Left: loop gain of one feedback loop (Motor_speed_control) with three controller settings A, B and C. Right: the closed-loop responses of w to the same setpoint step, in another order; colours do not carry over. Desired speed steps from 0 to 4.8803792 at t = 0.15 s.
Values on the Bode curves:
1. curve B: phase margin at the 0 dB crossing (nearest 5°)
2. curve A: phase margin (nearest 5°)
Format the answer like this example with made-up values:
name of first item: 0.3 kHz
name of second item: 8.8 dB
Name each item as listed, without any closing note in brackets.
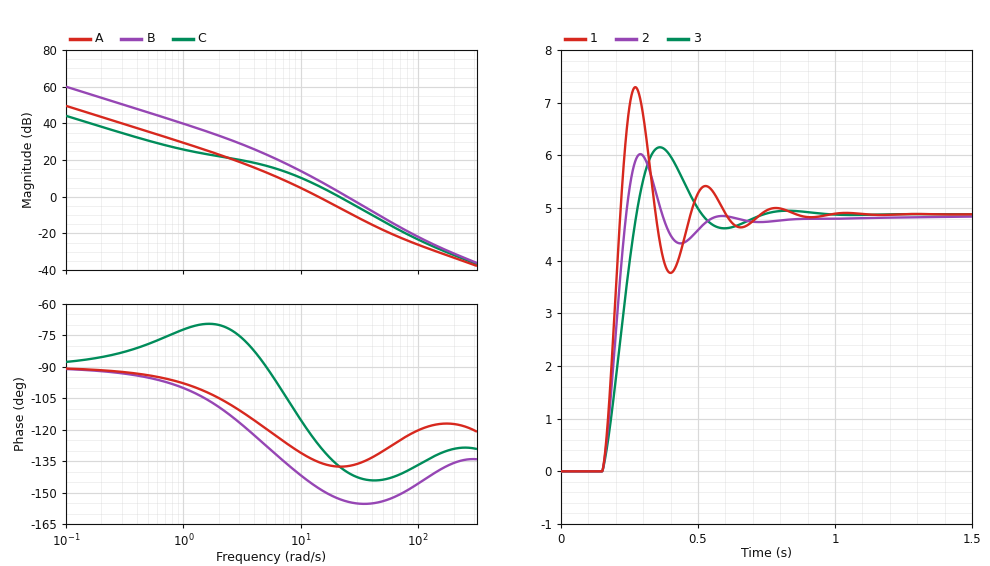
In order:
curve B: phase margin at the 0 dB crossing: 25°
curve A: phase margin: 45°
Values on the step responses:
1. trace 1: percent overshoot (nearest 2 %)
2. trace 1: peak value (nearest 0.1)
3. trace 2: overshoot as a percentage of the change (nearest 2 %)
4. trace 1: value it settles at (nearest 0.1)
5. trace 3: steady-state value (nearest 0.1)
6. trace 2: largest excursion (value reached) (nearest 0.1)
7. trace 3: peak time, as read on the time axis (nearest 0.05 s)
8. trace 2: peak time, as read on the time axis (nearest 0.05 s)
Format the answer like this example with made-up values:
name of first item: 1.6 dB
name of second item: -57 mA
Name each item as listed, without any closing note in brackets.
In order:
trace 1: percent overshoot: 50 %
trace 1: peak value: 7.3
trace 2: overshoot as a percentage of the change: 24 %
trace 1: value it settles at: 4.9
trace 3: steady-state value: 4.9
trace 2: largest excursion (value reached): 6.0
trace 3: peak time, as read on the time axis: 0.35 s
trace 2: peak time, as read on the time axis: 0.30 s
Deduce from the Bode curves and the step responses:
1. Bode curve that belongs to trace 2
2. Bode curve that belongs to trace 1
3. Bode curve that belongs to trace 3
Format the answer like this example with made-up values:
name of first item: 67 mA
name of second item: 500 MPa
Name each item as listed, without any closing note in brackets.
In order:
Bode curve that belongs to trace 2: C
Bode curve that belongs to trace 1: B
Bode curve that belongs to trace 3: A
